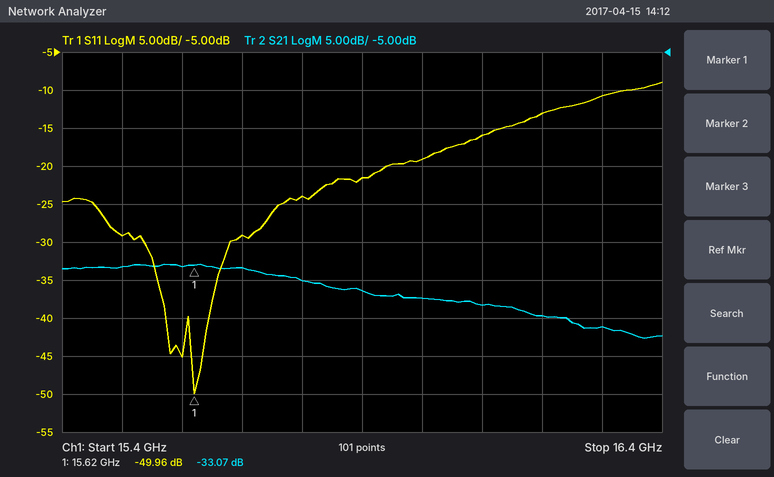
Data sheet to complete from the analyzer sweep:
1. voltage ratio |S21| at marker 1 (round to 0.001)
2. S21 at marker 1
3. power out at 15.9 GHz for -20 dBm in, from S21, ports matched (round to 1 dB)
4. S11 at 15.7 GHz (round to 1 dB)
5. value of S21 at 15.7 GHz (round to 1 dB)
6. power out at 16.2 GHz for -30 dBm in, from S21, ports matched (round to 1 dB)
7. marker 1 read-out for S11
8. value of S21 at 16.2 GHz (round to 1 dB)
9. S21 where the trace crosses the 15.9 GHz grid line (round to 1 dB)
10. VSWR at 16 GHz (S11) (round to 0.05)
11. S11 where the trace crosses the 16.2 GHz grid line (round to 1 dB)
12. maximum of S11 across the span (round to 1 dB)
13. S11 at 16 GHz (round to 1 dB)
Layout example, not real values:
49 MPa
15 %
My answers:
0.022
-33.07 dB
-56 dBm
-29 dB
-33 dB
-70 dBm
-49.96 dB
-40 dB
-36 dB
1.25
-13 dB
-9 dB
-19 dB
